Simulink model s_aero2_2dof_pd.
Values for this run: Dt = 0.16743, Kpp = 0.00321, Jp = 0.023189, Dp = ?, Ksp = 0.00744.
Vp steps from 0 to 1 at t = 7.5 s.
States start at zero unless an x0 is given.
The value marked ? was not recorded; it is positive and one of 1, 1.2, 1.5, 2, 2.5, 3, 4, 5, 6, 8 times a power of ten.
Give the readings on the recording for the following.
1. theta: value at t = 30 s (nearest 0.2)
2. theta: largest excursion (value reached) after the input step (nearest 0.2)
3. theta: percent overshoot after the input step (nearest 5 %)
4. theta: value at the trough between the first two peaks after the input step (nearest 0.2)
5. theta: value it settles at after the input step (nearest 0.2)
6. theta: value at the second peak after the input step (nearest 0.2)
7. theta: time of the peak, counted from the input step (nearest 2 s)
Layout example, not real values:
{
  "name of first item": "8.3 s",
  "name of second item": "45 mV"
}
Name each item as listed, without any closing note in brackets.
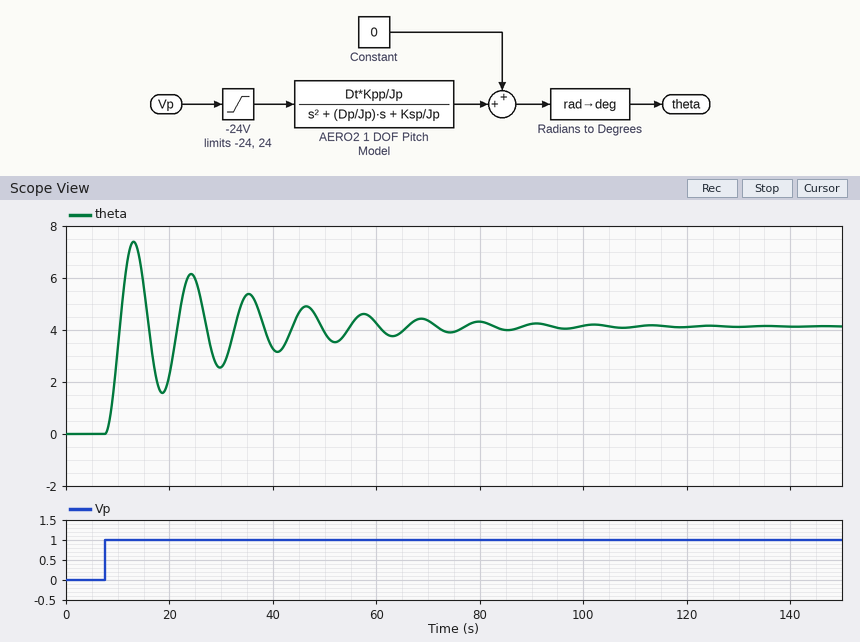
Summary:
{
  "theta: value at t = 30 s": "2.6",
  "theta: largest excursion (value reached) after the input step": "7.4",
  "theta: percent overshoot after the input step": "80 %",
  "theta: value at the trough between the first two peaks after the input step": "1.6",
  "theta: value it settles at after the input step": "4.2",
  "theta: value at the second peak after the input step": "6.2",
  "theta: time of the peak, counted from the input step": "6 s"
}
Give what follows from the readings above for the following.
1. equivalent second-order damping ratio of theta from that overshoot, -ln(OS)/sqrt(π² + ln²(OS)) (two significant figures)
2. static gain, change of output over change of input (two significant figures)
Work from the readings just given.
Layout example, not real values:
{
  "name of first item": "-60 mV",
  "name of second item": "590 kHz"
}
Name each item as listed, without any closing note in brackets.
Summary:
{
  "equivalent second-order damping ratio of theta from that overshoot, -ln(OS)/sqrt(π² + ln²(OS))": "0.071",
  "static gain, change of output over change of input": "4.2"
}
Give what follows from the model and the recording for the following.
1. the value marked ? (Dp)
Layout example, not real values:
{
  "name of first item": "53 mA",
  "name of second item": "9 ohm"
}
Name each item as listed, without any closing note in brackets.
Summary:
{
  "the value marked ?": "0.002"
}
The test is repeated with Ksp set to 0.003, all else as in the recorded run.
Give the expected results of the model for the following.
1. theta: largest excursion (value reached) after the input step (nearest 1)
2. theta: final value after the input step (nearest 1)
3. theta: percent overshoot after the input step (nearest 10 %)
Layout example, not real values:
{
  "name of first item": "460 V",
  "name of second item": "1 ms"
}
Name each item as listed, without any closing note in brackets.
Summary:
{
  "theta: largest excursion (value reached) after the input step": "17",
  "theta: final value after the input step": "10",
  "theta: percent overshoot after the input step": "70 %"
}
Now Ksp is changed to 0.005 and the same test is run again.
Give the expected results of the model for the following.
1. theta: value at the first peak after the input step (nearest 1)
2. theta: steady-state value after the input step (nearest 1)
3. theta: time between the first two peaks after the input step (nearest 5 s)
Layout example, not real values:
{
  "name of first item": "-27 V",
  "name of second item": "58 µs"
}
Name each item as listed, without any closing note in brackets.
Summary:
{
  "theta: value at the first peak after the input step": "11",
  "theta: steady-state value after the input step": "6",
  "theta: time between the first two peaks after the input step": "15 s"
}
